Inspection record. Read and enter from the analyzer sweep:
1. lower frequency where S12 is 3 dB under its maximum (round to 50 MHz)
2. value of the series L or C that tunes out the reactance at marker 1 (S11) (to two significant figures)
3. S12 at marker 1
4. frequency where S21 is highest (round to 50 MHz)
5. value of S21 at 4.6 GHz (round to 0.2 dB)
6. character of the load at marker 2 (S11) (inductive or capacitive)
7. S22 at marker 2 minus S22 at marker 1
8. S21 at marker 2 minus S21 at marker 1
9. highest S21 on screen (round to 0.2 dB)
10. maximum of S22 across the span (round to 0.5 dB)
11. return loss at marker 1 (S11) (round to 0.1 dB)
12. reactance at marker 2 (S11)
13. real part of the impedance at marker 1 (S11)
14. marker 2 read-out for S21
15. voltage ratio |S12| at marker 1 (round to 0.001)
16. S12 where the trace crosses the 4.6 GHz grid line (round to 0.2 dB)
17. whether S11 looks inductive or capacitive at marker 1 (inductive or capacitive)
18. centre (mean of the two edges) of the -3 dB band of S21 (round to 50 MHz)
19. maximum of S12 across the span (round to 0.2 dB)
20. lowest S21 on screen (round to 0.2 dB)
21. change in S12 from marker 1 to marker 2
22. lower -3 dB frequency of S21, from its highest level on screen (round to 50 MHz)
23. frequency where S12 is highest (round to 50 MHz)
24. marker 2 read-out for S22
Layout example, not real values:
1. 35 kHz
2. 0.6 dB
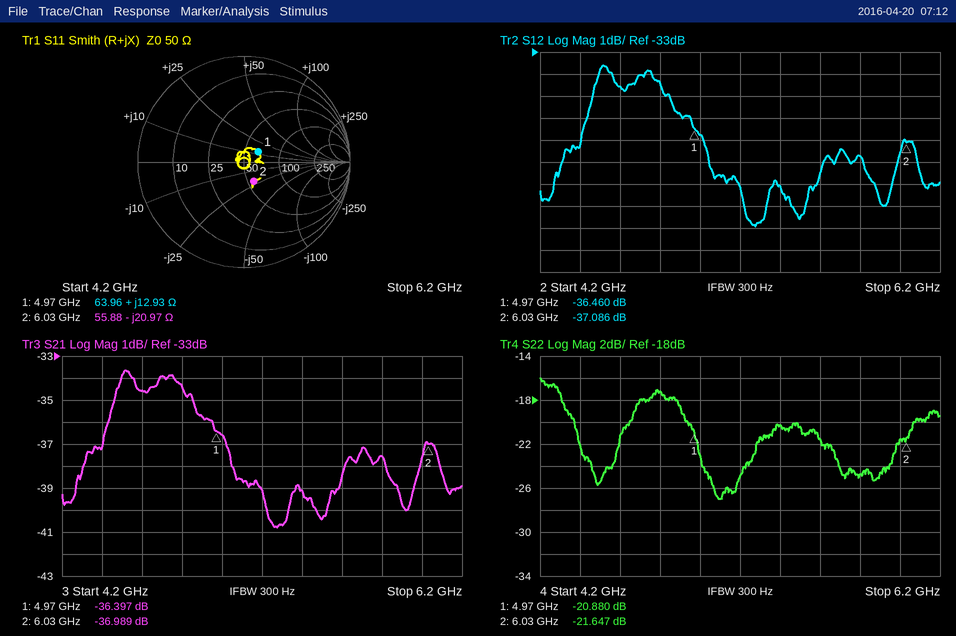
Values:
1. 4.40 GHz
2. 2.5 pF
3. -36.460 dB
4. 4.50 GHz
5. -34.6 dB
6. capacitive
7. -0.767 dB
8. -0.592 dB
9. -33.6 dB
10. -16.0 dB
11. 15.6 dB
12. -20.97 Ω
13. 63.96 Ω
14. -36.989 dB
15. 0.015
16. -34.6 dB
17. inductive
18. 4.70 GHz
19. -33.6 dB
20. -40.8 dB
21. -0.626 dB
22. 4.40 GHz
23. 4.50 GHz
24. -21.647 dB
